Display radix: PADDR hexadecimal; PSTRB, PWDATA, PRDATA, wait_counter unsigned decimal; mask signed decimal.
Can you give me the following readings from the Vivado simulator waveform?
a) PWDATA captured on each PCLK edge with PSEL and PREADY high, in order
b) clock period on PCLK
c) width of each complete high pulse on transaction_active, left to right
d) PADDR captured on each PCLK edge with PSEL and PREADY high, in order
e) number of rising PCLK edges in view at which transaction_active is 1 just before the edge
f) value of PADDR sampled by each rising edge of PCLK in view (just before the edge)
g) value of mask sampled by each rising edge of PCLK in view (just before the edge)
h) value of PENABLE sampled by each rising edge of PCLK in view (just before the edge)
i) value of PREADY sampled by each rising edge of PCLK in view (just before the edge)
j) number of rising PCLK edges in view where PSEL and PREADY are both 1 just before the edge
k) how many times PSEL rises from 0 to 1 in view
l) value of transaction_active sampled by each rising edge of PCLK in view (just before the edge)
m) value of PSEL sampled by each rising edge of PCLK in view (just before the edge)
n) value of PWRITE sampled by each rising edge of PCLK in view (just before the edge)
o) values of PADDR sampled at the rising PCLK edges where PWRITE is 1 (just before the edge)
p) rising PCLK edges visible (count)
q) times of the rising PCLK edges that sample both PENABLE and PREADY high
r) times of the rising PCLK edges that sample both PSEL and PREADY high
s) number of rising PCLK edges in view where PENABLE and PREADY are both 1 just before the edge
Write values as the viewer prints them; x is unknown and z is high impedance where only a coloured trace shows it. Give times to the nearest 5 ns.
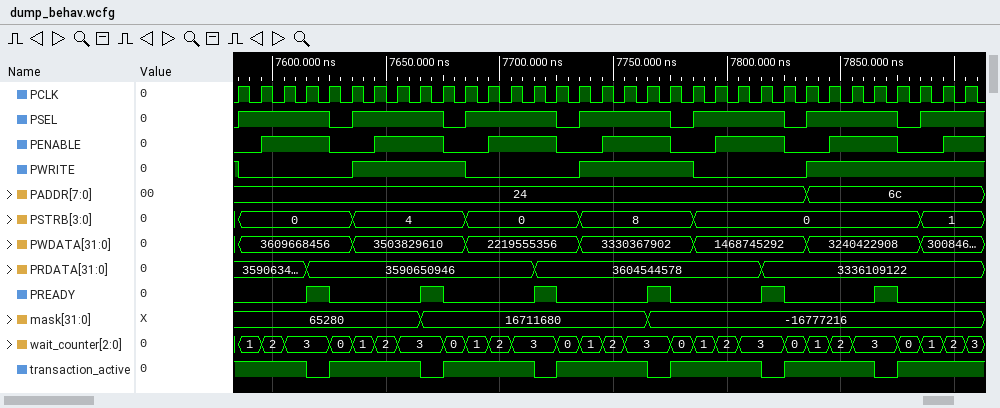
3609668456, 3503829610, 2219555356, 3330367902, 1468745292, 3240422908
10 ns
40 ns, 40 ns, 40 ns, 40 ns, 40 ns
24, 24, 24, 24, 24, 6c
27
24, 24, 24, 24, 24, 24, 24, 24, 24, 24, 24, 24, 24, 24, 24, 24, 24, 24, 24, 24, 24, 24, 24, 24, 24, 24, 6c, 6c, 6c, 6c, 6c, 6c, 6c
65280, 65280, 65280, 65280, 65280, 65280, 65280, 65280, 65280, 16711680, 16711680, 16711680, 16711680, 16711680, 16711680, 16711680, 16711680, 16711680, 16711680, -16777216, -16777216, -16777216, -16777216, -16777216, -16777216, -16777216, -16777216, -16777216, -16777216, -16777216, -16777216, -16777216, -16777216
0 0 1 1 1 0 0 1 1 1 0 0 1 1 1 0 0 1 1 1 0 0 1 1 1 0 0 1 1 1 0 0 1
0 0 0 0 1 0 0 0 0 1 0 0 0 0 1 0 0 0 0 1 0 0 0 0 1 0 0 0 0 1 0 0 0
6
7
1 1 1 1 0 1 1 1 1 0 1 1 1 1 0 1 1 1 1 0 1 1 1 1 0 1 1 1 1 0 1 1 1
0 1 1 1 1 0 1 1 1 1 0 1 1 1 1 0 1 1 1 1 0 1 1 1 1 0 1 1 1 1 0 1 1
1 0 0 0 0 0 1 1 1 1 1 0 0 0 0 0 1 1 1 1 1 0 0 0 0 0 1 1 1 1 1 1 1
24, 24, 24, 24, 24, 24, 24, 24, 24, 24, 24, 6c, 6c, 6c, 6c, 6c, 6c, 6c
33
7625 ns, 7675 ns, 7725 ns, 7775 ns, 7825 ns, 7875 ns
7625 ns, 7675 ns, 7725 ns, 7775 ns, 7825 ns, 7875 ns
6
